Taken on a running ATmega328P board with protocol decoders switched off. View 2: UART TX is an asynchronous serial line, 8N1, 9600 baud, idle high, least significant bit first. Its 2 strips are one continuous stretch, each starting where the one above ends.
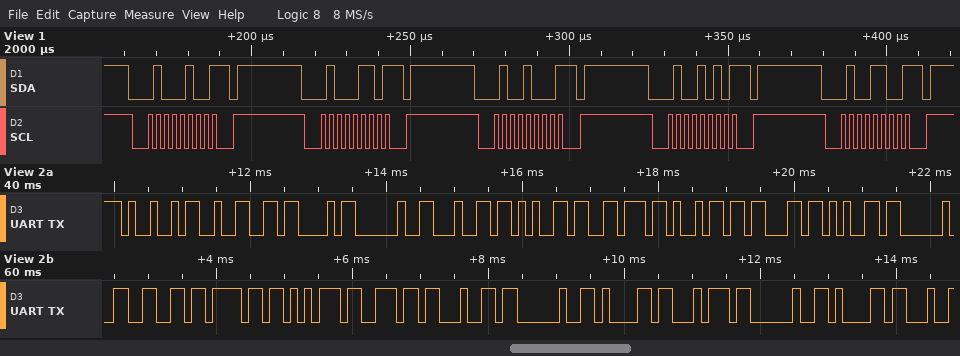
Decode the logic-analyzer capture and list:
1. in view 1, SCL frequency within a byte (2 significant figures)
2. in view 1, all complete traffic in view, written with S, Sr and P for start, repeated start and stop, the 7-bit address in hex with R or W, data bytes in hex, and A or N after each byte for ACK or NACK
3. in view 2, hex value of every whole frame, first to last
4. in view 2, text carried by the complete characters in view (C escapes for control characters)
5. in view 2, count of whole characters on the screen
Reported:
400 kHz
S 22W N P S 23W N P S 24W N P S 25W N P S 26W N P
49 32 43 20 64 65 76 69 63 65 20 66 6F 75 6E 64 20 61 74 20 61
"I2C device found at a"
21
